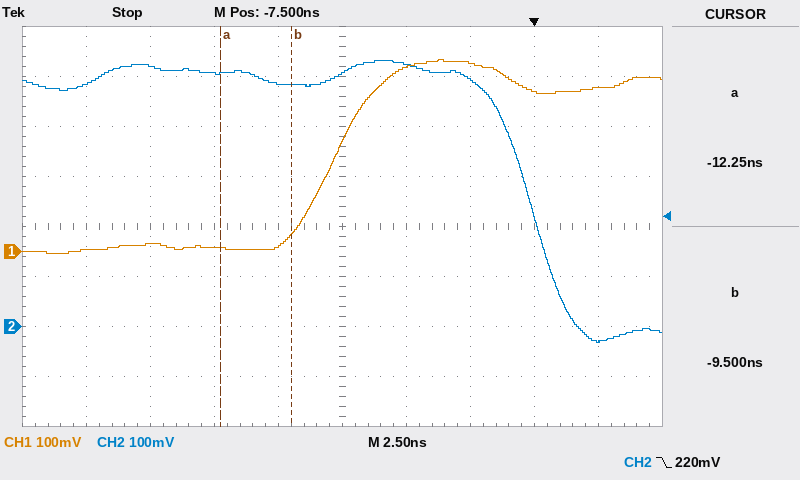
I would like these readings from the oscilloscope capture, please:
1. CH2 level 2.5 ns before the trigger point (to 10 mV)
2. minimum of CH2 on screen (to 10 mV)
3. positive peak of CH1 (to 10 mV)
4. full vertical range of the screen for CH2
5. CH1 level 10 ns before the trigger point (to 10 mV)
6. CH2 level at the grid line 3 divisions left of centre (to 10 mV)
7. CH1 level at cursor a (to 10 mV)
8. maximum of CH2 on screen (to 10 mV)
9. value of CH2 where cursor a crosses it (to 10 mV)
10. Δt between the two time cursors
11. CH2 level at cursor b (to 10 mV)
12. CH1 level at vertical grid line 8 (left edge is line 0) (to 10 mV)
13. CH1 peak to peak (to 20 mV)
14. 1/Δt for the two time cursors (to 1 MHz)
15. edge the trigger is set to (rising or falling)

490 mV
-30 mV
380 mV
800 mV
10 mV
520 mV
10 mV
530 mV
510 mV
2.75 ns
480 mV
320 mV
380 mV
364 MHz
falling
